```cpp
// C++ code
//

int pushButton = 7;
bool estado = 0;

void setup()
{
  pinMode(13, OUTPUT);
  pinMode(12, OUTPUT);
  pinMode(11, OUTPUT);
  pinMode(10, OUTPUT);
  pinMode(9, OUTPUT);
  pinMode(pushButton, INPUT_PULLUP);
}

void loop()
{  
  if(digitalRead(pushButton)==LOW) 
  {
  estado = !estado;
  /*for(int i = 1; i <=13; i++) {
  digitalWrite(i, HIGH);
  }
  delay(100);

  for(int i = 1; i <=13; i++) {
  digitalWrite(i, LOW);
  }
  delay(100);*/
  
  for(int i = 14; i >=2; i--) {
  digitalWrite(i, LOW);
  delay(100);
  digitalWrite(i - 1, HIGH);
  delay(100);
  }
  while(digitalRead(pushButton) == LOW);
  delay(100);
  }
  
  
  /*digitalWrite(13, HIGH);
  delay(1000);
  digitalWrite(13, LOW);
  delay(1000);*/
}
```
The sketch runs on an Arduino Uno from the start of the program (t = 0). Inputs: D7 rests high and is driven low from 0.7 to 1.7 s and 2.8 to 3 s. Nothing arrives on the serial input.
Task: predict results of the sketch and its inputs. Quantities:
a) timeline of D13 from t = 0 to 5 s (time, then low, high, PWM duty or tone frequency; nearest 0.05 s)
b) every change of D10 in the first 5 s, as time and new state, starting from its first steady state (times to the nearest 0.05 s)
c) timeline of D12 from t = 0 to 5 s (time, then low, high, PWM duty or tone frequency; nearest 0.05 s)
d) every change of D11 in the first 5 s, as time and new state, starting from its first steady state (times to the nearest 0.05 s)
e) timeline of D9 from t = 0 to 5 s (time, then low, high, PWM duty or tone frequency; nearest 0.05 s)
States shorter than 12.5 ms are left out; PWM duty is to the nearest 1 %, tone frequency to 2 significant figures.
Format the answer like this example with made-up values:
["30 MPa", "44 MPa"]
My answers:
["0 s low; 0.8 s high; 0.9 s low", "0 s low; 1.4 s high; 1.5 s low", "0 s low; 1 s high; 1.1 s low", "0 s low; 1.2 s high; 1.3 s low", "0 s low; 1.6 s high; 1.7 s low"]
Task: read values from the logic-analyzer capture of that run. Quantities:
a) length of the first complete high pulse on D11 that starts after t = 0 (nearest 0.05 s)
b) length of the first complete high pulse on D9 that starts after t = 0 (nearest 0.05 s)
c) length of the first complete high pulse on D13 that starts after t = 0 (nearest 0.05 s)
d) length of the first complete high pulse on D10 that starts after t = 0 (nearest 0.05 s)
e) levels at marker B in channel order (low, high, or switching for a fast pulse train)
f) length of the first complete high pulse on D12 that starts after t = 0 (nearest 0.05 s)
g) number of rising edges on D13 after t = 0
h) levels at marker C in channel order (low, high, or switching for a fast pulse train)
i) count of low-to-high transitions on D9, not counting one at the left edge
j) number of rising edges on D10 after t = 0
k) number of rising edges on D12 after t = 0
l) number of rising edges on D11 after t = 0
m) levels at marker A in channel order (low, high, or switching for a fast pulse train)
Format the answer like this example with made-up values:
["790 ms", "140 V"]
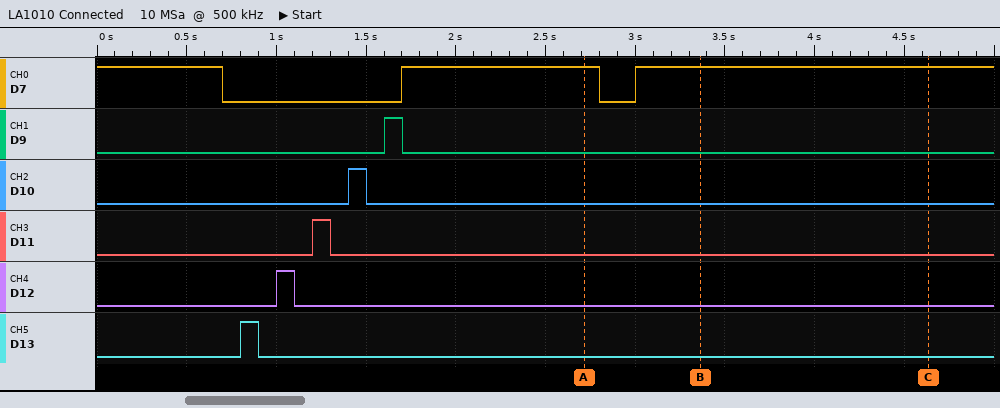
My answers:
["0.10 s", "0.10 s", "0.10 s", "0.10 s", "D7 high, D9 low, D10 low, D11 low, D12 low, D13 low", "0.10 s", "1", "D7 high, D9 low, D10 low, D11 low, D12 low, D13 low", "1", "1", "1", "1", "D7 high, D9 low, D10 low, D11 low, D12 low, D13 low"]
